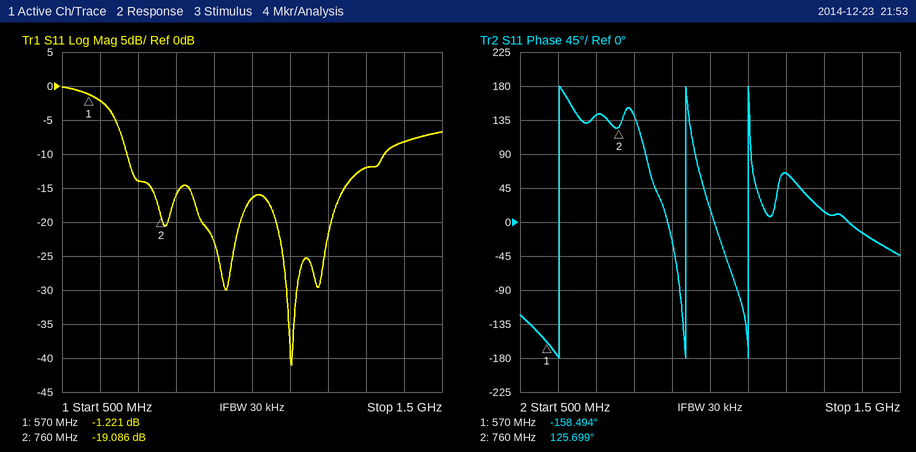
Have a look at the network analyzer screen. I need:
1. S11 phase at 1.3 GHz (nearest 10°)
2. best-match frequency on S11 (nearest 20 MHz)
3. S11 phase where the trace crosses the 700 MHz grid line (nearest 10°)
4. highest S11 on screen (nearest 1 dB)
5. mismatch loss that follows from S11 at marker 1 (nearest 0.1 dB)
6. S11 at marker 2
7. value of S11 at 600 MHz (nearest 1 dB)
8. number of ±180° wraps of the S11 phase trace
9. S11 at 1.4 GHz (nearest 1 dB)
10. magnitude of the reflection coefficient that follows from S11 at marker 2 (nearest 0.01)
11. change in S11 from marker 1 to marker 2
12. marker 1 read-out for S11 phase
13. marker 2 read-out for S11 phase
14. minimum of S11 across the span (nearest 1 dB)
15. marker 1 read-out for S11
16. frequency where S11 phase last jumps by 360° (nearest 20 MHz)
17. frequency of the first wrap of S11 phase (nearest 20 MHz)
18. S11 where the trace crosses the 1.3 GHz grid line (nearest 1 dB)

10°
1.10 GHz
140°
0 dB
6.1 dB
-19.086 dB
-2 dB
3
-8 dB
0.11
-17.865 dB
-158.494°
125.699°
-41 dB
-1.221 dB
1.10 GHz
600 MHz
-12 dB
